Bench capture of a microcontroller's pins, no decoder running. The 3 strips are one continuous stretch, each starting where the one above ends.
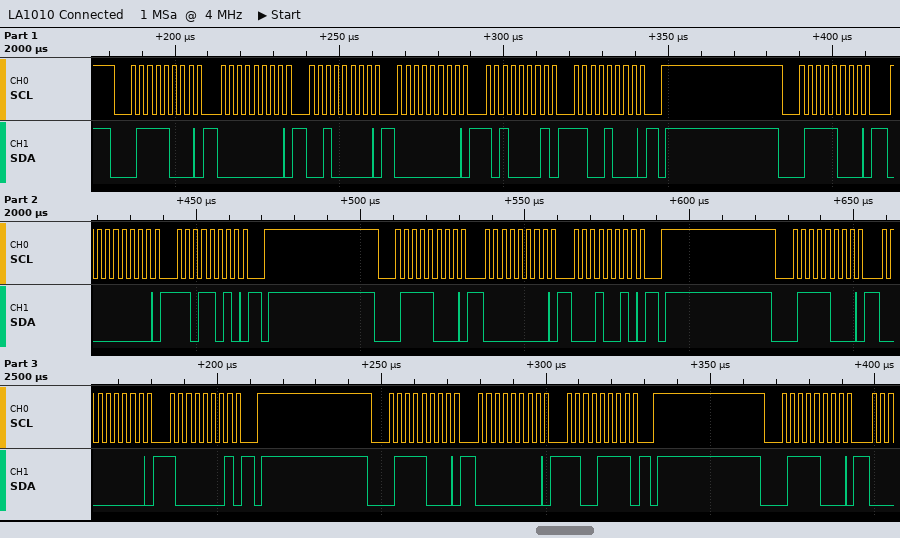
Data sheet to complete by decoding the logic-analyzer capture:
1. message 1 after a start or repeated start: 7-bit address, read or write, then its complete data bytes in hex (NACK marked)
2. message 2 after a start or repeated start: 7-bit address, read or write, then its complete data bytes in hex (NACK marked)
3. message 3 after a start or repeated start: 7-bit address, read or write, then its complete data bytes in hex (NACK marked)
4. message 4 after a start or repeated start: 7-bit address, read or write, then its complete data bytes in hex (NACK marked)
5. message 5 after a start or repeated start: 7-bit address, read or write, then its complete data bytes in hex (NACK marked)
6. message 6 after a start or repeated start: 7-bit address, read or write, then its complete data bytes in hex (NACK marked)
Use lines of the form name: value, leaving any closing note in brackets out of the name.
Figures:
message 1 after a start or repeated start: 7-bit address, read or write, then its complete data bytes in hex: 0x3C write: 00 20 00 A1 C8
message 2 after a start or repeated start: 7-bit address, read or write, then its complete data bytes in hex: 0x3C write: 00 DA
message 3 after a start or repeated start: 7-bit address, read or write, then its complete data bytes in hex: 0x3C write: 00 12
message 4 after a start or repeated start: 7-bit address, read or write, then its complete data bytes in hex: 0x3C write: 00 81
message 5 after a start or repeated start: 7-bit address, read or write, then its complete data bytes in hex: 0x3C write: 00 CF
message 6 after a start or repeated start: 7-bit address, read or write, then its complete data bytes in hex: 0x3C write
